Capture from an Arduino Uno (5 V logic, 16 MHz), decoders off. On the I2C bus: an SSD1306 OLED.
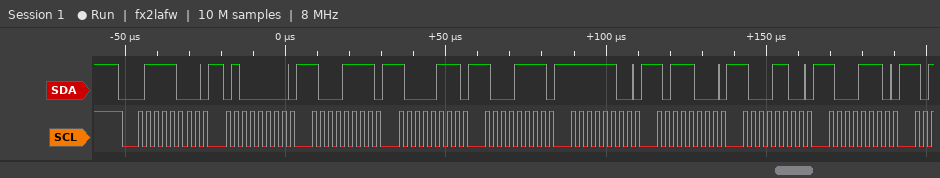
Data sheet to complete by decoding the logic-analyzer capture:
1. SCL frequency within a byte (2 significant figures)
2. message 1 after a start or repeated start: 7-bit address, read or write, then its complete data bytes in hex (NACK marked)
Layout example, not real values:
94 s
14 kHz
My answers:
400 kHz
0x3C write: 40 8F 87 8F FC B8 8C 8E
